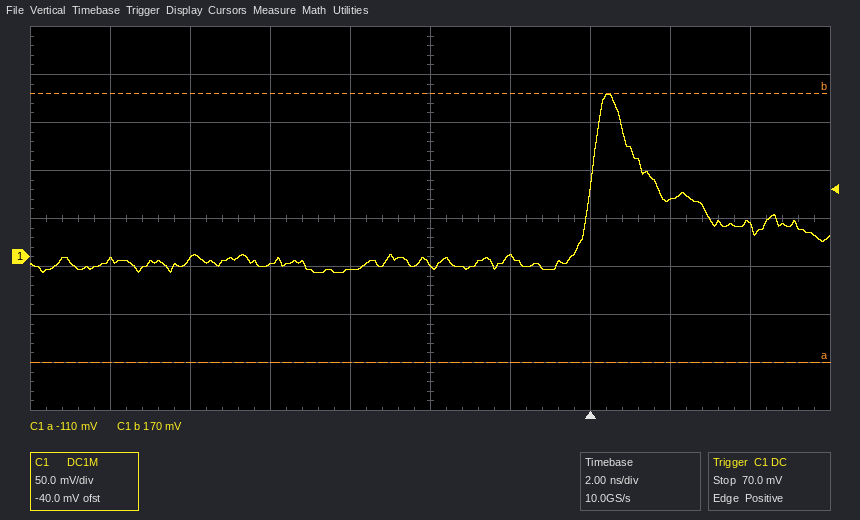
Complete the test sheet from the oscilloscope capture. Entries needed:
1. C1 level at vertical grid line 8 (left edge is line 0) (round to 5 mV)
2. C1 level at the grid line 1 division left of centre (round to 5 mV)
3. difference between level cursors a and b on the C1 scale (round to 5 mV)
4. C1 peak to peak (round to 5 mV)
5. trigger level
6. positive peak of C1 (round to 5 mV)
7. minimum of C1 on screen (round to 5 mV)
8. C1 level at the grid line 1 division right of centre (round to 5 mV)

60 mV
-15 mV
280 mV
185 mV
70.0 mV
170 mV
-15 mV
0 mV
